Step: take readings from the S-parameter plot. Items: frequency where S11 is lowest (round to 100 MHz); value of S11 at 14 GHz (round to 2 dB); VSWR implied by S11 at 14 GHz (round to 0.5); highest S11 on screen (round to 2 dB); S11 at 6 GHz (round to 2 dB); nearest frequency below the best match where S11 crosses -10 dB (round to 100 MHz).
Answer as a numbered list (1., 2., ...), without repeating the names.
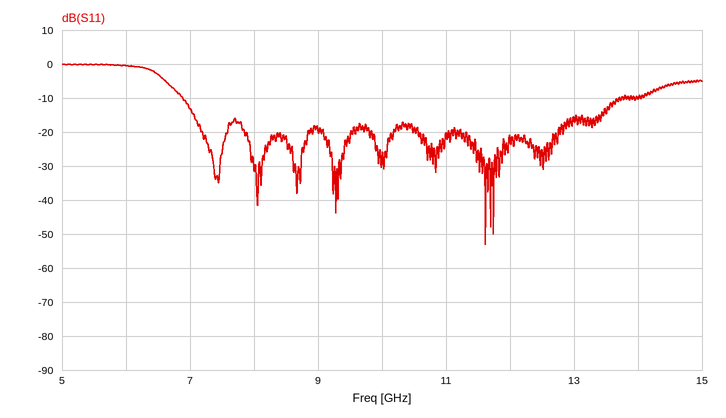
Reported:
1. 11.6 GHz
2. -10 dB
3. 2.0
4. 0 dB
5. 0 dB
6. 6.9 GHz
